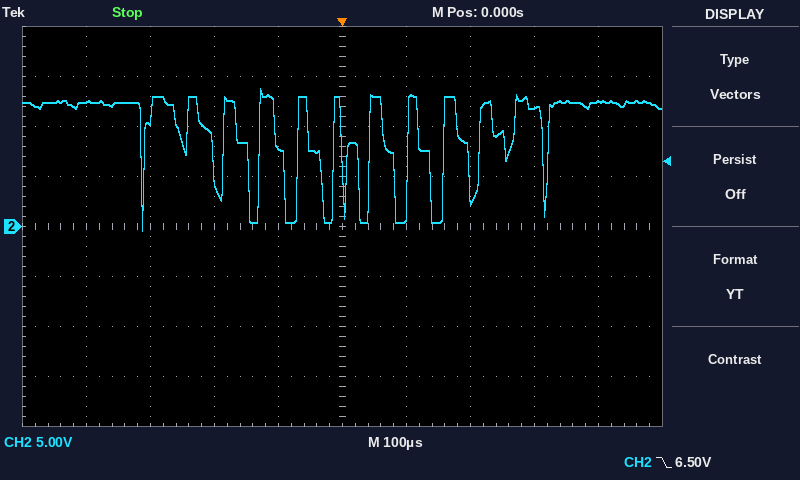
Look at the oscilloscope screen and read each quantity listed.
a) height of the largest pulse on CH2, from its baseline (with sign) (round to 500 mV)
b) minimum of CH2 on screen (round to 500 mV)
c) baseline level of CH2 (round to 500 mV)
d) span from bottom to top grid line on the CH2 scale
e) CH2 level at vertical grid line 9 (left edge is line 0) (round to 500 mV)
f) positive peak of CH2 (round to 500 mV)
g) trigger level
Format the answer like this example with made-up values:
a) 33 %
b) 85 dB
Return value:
a) -13.0 V
b) -500 mV
c) 12.5 V
d) 40 V
e) 12.5 V
f) 14.0 V
g) 6.50 V
